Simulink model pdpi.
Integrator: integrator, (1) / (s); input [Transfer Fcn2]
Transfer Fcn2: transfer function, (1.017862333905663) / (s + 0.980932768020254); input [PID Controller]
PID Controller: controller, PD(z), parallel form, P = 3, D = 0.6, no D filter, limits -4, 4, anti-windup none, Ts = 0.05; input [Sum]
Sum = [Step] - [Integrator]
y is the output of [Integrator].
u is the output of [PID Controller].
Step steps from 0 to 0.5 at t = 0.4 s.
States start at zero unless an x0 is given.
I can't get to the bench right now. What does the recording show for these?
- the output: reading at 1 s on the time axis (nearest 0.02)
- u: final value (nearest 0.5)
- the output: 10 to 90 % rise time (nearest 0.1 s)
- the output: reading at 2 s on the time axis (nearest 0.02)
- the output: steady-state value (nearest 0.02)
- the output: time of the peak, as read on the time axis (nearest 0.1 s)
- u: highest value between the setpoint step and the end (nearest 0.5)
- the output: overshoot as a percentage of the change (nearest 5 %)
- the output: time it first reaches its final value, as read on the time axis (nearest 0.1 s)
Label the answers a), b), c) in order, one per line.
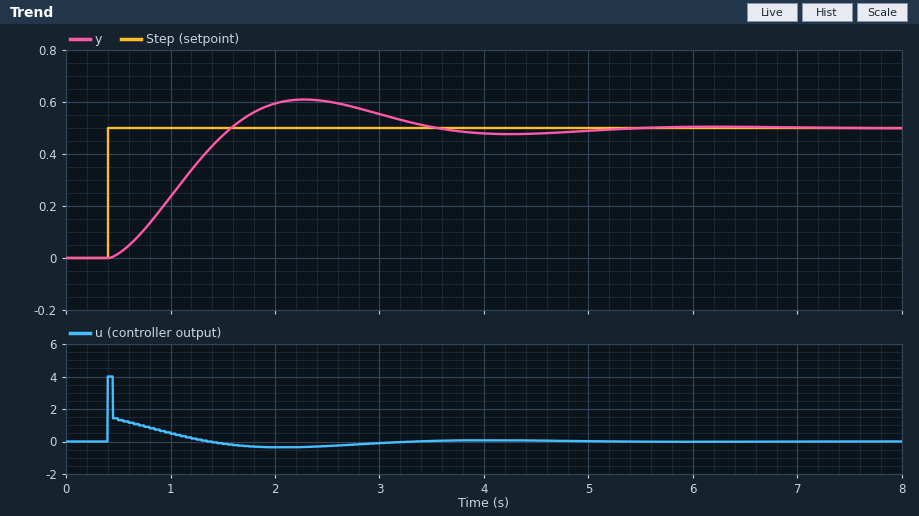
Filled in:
a) 0.24
b) 0.0
c) 0.8 s
d) 0.60
e) 0.50
f) 2.3 s
g) 4.0
h) 20 %
i) 1.6 s
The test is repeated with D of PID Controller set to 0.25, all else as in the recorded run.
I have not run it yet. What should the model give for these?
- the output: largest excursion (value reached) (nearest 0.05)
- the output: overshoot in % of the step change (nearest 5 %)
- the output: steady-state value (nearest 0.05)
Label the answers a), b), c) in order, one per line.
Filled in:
a) 0.65
b) 35 %
c) 0.50
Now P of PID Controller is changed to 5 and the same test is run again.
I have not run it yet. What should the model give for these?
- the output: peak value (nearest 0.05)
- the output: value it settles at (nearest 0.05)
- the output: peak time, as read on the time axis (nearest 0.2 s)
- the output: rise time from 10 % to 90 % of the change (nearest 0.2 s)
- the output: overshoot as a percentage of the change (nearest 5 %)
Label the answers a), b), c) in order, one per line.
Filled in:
a) 0.65
b) 0.50
c) 1.8 s
d) 0.6 s
e) 35 %
